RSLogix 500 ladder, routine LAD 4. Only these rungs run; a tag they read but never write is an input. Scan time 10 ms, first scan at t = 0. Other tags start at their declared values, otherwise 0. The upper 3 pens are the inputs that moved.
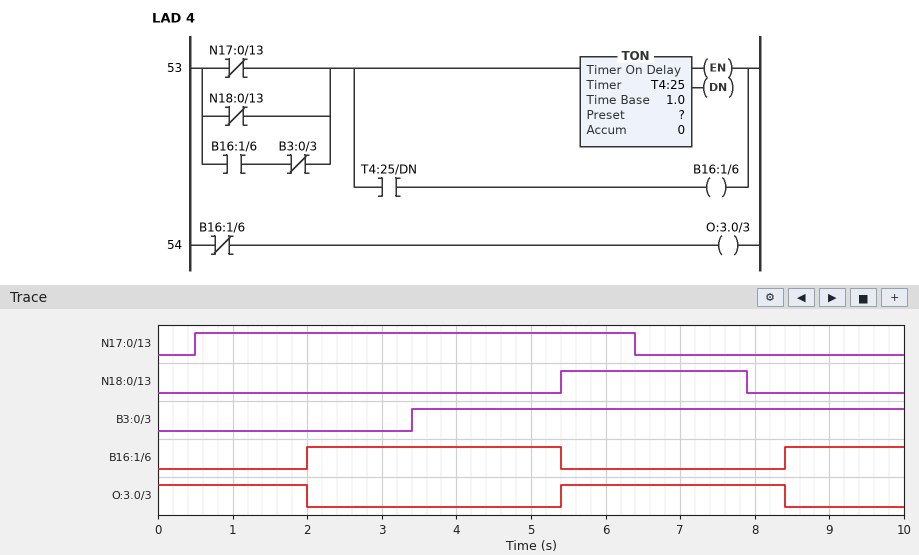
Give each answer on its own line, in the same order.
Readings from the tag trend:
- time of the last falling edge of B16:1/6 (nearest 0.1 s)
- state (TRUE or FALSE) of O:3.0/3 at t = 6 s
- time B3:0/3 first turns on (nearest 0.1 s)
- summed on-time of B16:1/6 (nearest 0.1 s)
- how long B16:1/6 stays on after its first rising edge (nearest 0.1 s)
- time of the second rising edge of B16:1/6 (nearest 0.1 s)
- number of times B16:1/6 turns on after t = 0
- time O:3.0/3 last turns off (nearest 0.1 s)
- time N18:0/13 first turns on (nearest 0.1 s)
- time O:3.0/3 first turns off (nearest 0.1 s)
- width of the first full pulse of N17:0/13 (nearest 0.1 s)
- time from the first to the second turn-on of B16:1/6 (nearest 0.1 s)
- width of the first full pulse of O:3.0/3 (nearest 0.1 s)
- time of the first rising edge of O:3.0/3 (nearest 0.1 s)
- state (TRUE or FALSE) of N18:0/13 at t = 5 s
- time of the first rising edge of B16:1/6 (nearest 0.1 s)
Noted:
5.4 s
TRUE
3.4 s
5.0 s
3.4 s
8.4 s
2
8.4 s
5.4 s
2.0 s
5.9 s
6.4 s
3.0 s
5.4 s
FALSE
2.0 s
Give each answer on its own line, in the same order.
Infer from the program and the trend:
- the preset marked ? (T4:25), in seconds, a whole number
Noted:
2 s
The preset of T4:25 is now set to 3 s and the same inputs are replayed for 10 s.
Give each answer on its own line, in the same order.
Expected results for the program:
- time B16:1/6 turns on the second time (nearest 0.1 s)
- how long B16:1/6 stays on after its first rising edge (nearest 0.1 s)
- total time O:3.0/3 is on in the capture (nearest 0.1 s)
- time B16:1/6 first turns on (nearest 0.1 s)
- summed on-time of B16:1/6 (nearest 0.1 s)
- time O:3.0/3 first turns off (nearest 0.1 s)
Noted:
9.4 s
2.4 s
7.0 s
3.0 s
3.0 s
3.0 s
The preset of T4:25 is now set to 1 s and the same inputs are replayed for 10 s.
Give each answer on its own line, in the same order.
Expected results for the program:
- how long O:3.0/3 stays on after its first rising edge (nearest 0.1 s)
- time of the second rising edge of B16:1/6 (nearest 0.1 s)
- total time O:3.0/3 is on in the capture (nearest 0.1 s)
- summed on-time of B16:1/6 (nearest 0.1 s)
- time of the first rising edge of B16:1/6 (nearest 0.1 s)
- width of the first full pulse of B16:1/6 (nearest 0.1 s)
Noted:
2.0 s
7.4 s
3.0 s
7.0 s
1.0 s
4.4 s
